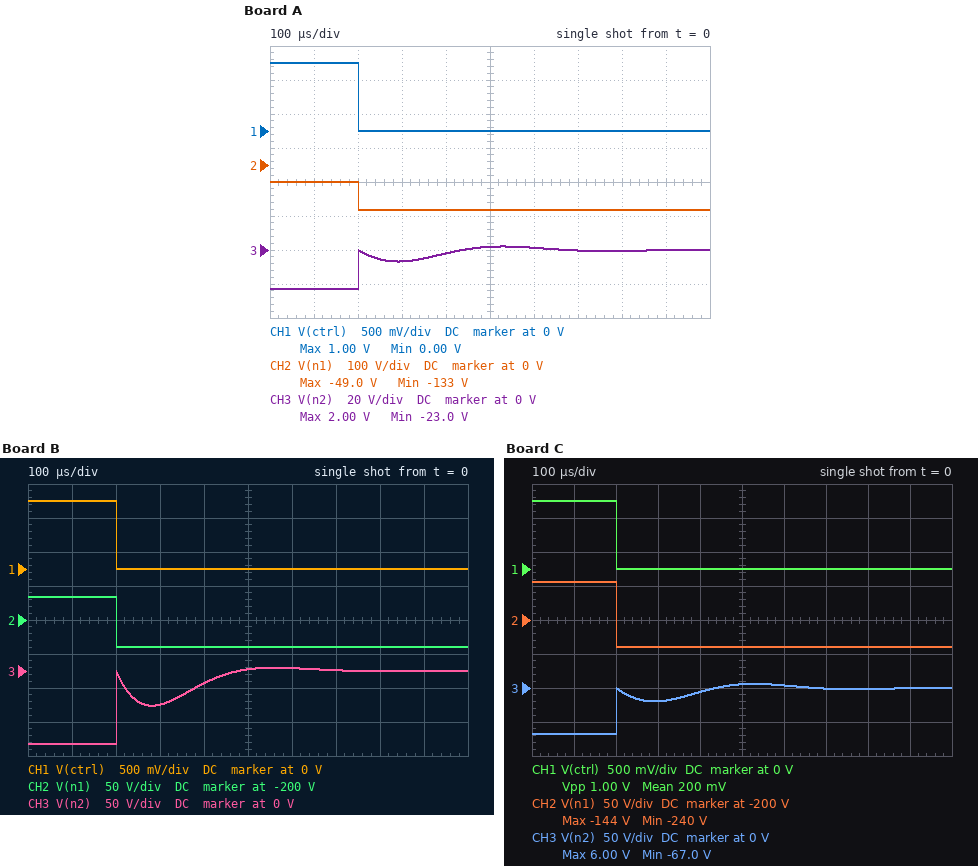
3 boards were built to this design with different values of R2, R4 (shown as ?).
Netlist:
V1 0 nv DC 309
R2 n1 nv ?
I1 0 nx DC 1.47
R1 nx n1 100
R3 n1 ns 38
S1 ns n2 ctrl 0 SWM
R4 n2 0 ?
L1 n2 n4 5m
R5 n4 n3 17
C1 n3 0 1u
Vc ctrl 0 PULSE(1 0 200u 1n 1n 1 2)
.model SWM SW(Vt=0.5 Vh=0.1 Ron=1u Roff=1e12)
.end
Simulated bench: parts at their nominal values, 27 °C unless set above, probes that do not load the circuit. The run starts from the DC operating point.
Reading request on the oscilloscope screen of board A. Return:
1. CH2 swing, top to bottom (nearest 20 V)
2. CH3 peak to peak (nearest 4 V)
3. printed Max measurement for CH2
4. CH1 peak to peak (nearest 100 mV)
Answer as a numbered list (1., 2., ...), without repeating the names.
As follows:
1. 80 V
2. 24 V
3. -49.0 V
4. 1.0 V
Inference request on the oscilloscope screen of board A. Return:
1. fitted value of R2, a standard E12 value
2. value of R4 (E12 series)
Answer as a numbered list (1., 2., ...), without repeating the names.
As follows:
1. 120 Ω
2. 33 Ω
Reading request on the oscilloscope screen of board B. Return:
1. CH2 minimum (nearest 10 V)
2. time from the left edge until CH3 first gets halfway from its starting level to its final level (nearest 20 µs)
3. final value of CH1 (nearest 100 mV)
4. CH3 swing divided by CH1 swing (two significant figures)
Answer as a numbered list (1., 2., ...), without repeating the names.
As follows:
1. -240 V
2. 200 µs
3. 0 V
4. 110
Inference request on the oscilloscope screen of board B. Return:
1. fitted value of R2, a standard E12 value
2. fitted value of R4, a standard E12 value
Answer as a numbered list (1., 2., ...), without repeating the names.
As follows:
1. 47 Ω
2. 68 Ω
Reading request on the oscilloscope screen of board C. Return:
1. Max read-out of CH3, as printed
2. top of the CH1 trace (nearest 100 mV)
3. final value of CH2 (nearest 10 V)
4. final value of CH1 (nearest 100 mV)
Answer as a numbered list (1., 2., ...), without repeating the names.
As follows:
1. 6.00 V
2. 1.0 V
3. -240 V
4. 0 V
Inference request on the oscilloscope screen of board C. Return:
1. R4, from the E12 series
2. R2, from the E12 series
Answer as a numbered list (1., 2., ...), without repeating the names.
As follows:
1. 33 Ω
2. 47 Ω
